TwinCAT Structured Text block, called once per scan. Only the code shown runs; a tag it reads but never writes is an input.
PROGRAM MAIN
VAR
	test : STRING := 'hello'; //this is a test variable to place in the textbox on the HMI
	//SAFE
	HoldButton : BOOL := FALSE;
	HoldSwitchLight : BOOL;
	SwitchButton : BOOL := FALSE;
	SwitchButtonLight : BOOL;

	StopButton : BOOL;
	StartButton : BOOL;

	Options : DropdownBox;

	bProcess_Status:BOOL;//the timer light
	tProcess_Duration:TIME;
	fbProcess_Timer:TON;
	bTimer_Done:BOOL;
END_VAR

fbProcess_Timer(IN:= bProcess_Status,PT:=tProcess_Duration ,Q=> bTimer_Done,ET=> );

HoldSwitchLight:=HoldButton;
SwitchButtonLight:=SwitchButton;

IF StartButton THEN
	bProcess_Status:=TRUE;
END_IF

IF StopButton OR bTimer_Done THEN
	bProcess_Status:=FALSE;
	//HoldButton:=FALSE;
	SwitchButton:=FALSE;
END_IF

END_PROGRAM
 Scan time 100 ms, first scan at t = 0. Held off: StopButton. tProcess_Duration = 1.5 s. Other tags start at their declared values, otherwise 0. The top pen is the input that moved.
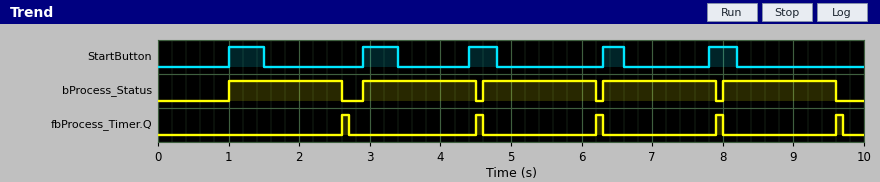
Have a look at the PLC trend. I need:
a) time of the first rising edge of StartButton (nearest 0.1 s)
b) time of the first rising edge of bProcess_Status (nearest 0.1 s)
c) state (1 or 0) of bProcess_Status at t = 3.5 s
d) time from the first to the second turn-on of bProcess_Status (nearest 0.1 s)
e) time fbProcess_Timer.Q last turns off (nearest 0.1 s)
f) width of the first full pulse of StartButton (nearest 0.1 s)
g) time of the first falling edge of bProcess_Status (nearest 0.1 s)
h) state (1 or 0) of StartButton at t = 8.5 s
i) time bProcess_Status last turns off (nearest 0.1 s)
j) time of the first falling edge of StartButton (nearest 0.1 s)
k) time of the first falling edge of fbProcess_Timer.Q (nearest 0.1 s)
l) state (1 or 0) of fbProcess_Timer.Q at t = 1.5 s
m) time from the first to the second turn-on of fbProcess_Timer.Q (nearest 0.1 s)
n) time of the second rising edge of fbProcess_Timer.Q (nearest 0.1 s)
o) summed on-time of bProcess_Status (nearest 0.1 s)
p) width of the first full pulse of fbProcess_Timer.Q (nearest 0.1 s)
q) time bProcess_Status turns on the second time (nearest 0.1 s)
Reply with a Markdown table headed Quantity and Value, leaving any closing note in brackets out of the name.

| Quantity | Value |
|---|---|
| time of the first rising edge of StartButton | 1.0 s |
| time of the first rising edge of bProcess_Status | 1.0 s |
| state (1 or 0) of bProcess_Status at t = 3.5 s | 1 |
| time from the first to the second turn-on of bProcess_Status | 1.9 s |
| time fbProcess_Timer.Q last turns off | 9.7 s |
| width of the first full pulse of StartButton | 0.5 s |
| time of the first falling edge of bProcess_Status | 2.6 s |
| state (1 or 0) of StartButton at t = 8.5 s | 0 |
| time bProcess_Status last turns off | 9.6 s |
| time of the first falling edge of StartButton | 1.5 s |
| time of the first falling edge of fbProcess_Timer.Q | 2.7 s |
| state (1 or 0) of fbProcess_Timer.Q at t = 1.5 s | 0 |
| time from the first to the second turn-on of fbProcess_Timer.Q | 1.9 s |
| time of the second rising edge of fbProcess_Timer.Q | 4.5 s |
| summed on-time of bProcess_Status | 8.0 s |
| width of the first full pulse of fbProcess_Timer.Q | 0.1 s |
| time bProcess_Status turns on the second time | 2.9 s |
